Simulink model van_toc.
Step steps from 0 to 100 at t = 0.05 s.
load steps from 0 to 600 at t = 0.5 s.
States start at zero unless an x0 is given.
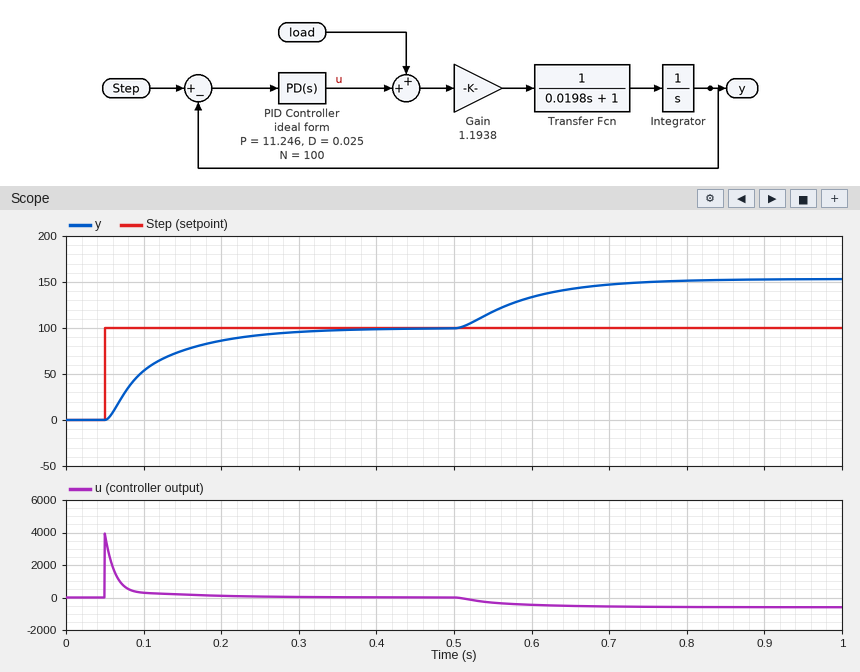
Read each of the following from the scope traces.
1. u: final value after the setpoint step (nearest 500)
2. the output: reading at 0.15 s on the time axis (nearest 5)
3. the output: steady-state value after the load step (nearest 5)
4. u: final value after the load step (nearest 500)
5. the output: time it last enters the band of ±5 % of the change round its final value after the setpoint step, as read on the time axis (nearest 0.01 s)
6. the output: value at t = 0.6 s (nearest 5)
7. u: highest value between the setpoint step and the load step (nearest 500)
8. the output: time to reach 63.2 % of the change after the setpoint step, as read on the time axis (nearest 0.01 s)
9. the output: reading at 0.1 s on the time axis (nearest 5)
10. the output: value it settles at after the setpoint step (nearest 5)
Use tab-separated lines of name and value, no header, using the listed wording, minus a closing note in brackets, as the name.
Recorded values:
u: final value after the setpoint step	0
the output: reading at 0.15 s on the time axis	75
the output: steady-state value after the load step	155
u: final value after the load step	-500
the output: time it last enters the band of ±5 % of the change round its final value after the setpoint step, as read on the time axis	0.29 s
the output: value at t = 0.6 s	135
u: highest value between the setpoint step and the load step	4000
the output: time to reach 63.2 % of the change after the setpoint step, as read on the time axis	0.12 s
the output: reading at 0.1 s on the time axis	55
the output: value it settles at after the setpoint step	100
